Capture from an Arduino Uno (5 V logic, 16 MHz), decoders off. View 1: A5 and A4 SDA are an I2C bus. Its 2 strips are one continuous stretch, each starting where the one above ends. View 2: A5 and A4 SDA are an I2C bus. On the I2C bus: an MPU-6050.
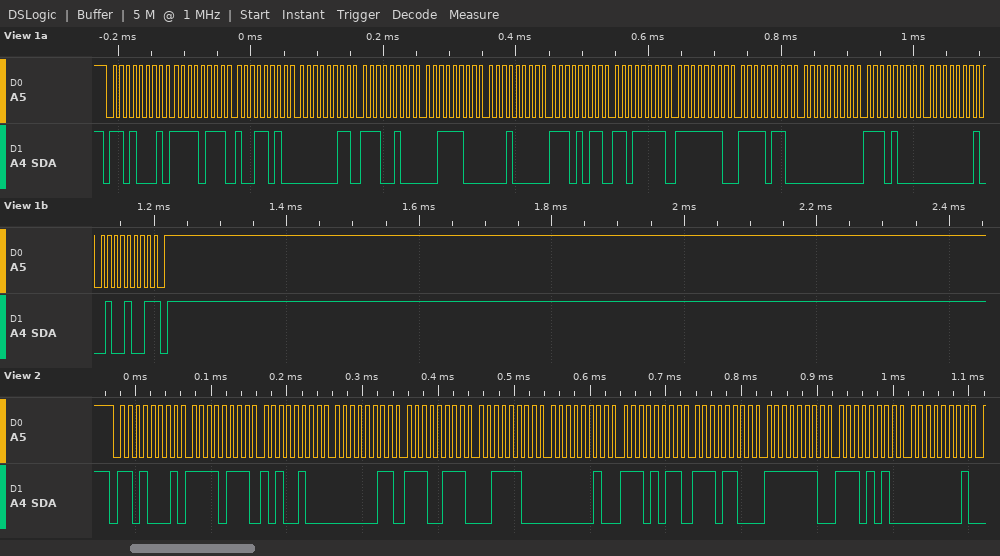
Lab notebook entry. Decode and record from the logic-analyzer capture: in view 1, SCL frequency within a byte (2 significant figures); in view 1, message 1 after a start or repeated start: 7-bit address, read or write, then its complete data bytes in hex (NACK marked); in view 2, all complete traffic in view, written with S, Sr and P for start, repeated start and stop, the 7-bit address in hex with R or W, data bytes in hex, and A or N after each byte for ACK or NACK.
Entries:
100 kHz
0x68 read: F7 9A 03 E4 3C 10 EB DF FE F6 00 E8 01 49 NACK
S 68R A F7 A A4 A 03 A E7 A 3C A 02 A EB A EC A FE A EA A 01 A
